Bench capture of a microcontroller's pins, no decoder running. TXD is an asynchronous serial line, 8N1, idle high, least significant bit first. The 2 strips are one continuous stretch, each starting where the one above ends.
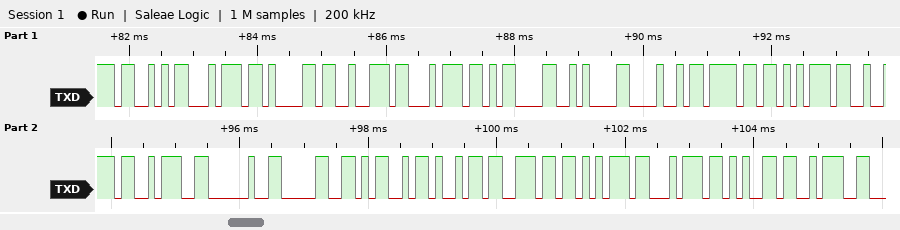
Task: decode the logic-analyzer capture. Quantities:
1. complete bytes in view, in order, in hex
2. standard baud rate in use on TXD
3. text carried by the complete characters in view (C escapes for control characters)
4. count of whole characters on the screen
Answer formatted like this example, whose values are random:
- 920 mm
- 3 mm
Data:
- 53 74 61 72 74 0D 0A 48 6F 75 72 3A 20 30 4D 69 6E 75 74 65 3A
- 9600 baud
- "Start\r\nHour: 0Minute:"
- 21
